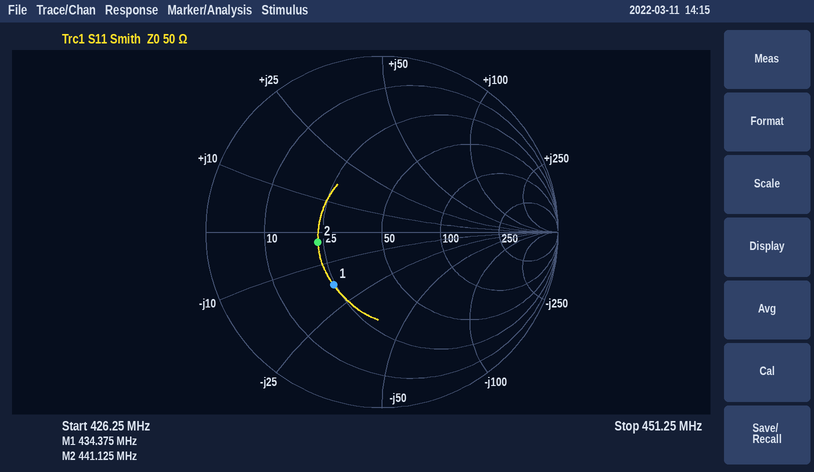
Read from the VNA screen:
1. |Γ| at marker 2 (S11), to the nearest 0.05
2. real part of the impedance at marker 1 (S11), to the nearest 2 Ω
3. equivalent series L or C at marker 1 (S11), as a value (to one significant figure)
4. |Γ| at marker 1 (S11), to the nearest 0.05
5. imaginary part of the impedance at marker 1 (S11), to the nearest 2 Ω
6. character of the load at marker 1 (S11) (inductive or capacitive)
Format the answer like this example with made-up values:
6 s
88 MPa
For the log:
0.35
24 Ω
20 pF
0.40
-18 Ω
capacitive
